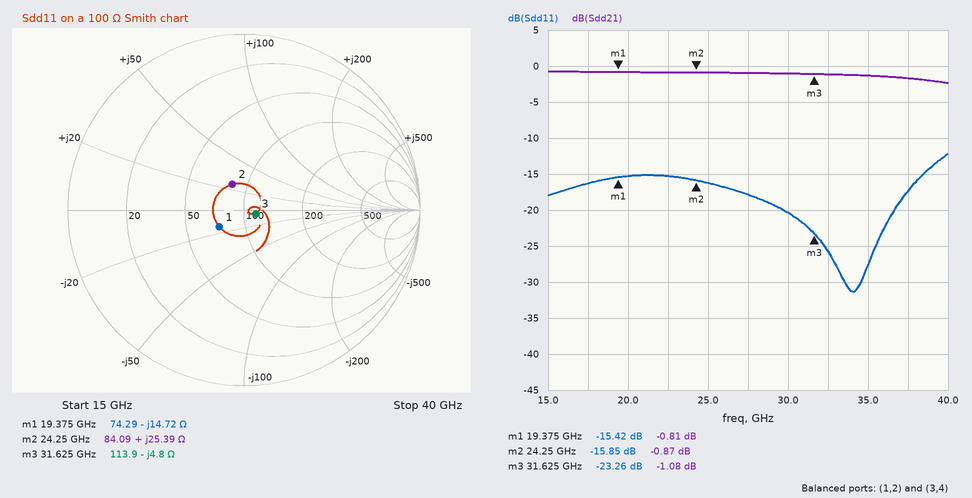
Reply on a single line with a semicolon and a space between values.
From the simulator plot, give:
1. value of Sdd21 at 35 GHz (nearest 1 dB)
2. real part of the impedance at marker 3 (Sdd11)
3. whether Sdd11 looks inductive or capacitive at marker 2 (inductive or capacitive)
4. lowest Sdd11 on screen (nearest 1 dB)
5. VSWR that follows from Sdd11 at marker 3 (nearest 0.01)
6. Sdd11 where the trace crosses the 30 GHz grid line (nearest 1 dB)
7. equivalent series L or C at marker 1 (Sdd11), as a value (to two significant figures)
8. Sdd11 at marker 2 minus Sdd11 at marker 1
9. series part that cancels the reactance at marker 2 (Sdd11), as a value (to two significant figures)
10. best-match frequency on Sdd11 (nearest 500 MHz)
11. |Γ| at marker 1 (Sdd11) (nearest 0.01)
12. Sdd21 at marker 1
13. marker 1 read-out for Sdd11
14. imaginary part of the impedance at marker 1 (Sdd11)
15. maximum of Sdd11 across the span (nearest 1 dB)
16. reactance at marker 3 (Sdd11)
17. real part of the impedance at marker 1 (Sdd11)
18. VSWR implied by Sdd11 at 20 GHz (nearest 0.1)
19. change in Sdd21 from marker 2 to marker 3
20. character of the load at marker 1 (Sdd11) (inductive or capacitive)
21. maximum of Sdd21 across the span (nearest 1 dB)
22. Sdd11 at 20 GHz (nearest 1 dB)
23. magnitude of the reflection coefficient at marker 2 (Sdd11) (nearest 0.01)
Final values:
-1 dB; 113.9 Ω; inductive; -31 dB; 1.15; -20 dB; 560 fF; -0.43 dB; 260 fF; 34.0 GHz; 0.17; -0.81 dB; -15.42 dB; -14.72 Ω; -12 dB; -4.8 Ω; 74.29 Ω; 1.4; -0.21 dB; capacitive; -1 dB; -15 dB; 0.16
